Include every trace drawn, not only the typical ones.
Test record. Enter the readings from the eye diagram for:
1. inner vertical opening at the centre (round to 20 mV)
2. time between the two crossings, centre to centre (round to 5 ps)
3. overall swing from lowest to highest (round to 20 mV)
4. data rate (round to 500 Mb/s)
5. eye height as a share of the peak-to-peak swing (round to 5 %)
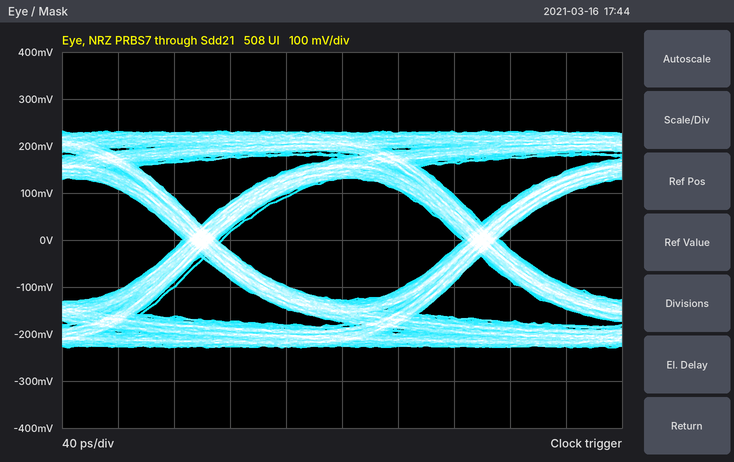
260 mV
200 ps
460 mV
5.0 Gb/s
55 %
